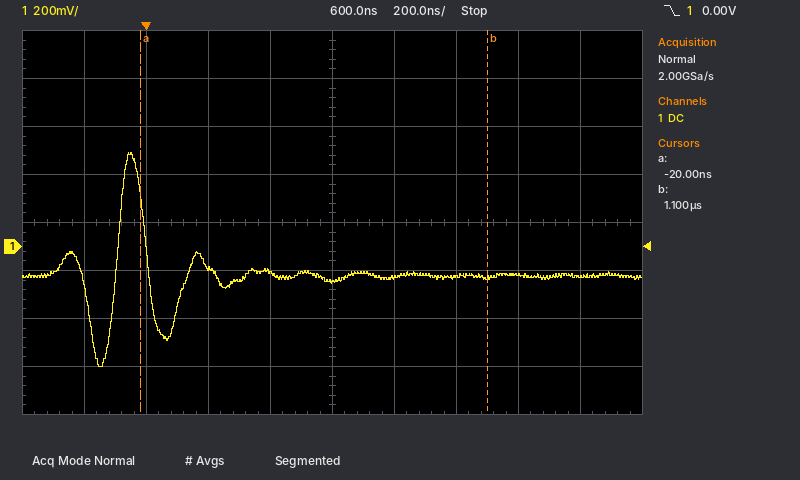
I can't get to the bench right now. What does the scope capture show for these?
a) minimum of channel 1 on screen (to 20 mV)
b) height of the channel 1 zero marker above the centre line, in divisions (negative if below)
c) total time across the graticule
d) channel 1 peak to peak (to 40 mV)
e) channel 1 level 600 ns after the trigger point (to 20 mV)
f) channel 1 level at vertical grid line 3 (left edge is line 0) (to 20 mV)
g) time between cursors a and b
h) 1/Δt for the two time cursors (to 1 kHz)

-500 mV
-0.5 div
2 µs
880 mV
-140 mV
-80 mV
1.12 µs
893 kHz
